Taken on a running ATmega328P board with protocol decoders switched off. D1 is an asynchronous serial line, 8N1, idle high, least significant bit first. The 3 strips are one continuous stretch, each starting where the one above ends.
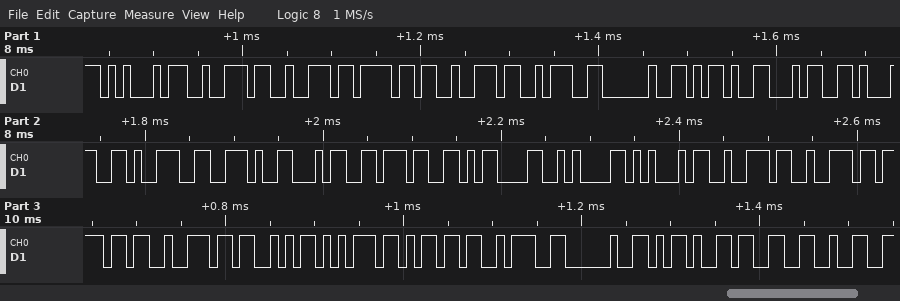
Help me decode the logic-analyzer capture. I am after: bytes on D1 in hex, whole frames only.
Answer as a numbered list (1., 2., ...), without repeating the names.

1. 45 72 72 6F 72 3A 20 2D 34 31 39 2E 34 37 0D 0A 45 72 72 6F 72 53 75 6D 3A 20 2D 33 32
